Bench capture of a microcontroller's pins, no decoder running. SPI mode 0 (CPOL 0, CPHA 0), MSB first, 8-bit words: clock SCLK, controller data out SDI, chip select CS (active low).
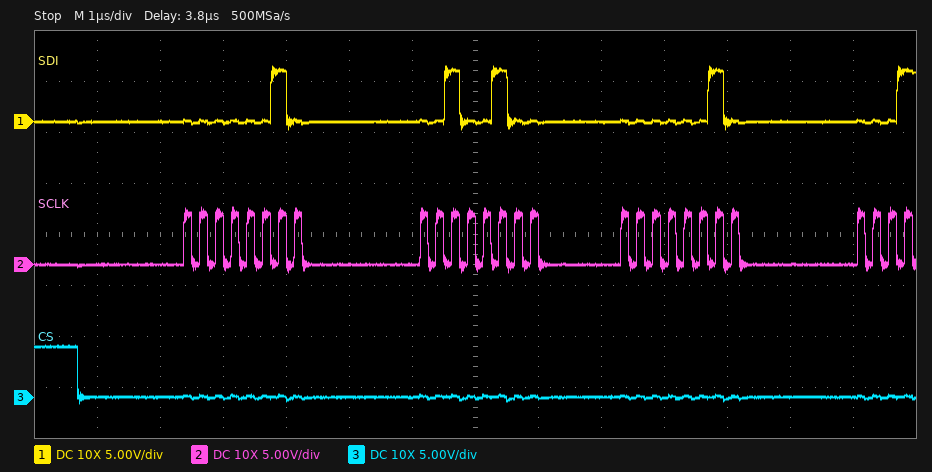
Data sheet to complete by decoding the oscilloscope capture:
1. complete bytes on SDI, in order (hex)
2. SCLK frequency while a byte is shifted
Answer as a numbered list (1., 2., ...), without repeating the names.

1. 02 24 02
2. 4 MHz
